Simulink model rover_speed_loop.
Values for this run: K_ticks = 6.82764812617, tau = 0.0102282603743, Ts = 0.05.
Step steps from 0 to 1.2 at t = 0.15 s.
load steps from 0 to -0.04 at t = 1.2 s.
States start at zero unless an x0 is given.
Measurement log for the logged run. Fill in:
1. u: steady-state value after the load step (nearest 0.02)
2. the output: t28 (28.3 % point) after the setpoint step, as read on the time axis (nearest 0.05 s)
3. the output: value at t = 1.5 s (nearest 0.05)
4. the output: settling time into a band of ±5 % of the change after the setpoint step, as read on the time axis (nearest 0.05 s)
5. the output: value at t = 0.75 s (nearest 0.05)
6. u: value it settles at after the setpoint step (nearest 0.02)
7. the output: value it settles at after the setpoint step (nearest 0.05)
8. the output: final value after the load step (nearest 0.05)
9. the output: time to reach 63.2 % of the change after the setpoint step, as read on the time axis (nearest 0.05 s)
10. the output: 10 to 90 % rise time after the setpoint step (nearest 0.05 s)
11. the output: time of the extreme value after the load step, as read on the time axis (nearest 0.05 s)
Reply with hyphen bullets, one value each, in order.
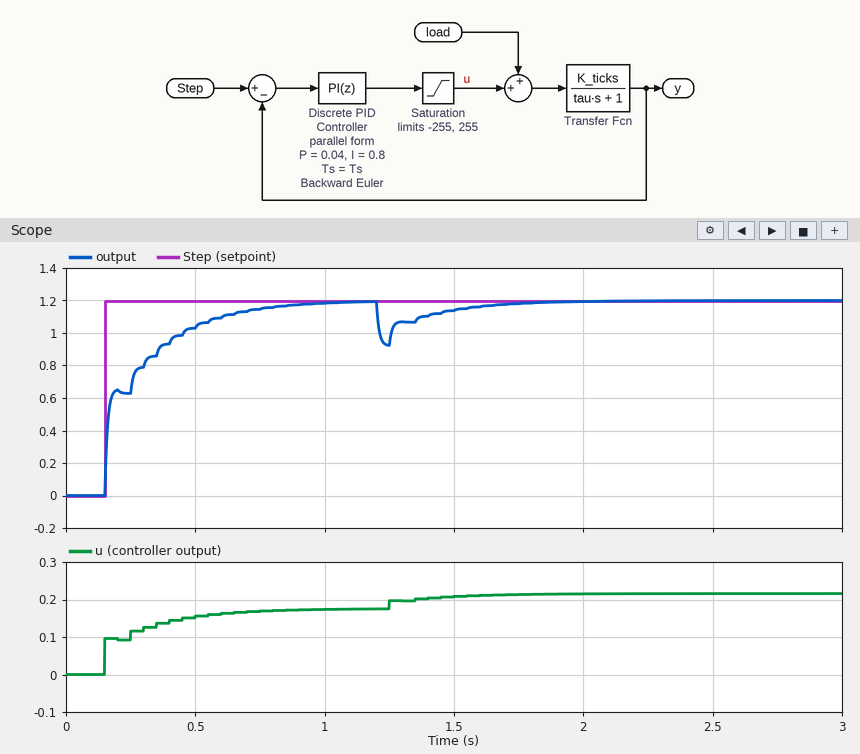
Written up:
- 0.22
- 0.15 s
- 1.15
- 0.70 s
- 1.15
- 0.18
- 1.20
- 1.20
- 0.25 s
- 0.40 s
- 1.25 s
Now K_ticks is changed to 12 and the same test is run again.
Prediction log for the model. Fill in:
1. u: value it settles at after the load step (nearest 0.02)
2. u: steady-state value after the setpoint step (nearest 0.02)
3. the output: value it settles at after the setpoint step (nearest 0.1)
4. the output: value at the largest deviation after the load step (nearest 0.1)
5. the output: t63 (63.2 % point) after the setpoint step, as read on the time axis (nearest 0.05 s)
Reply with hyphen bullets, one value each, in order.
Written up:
- 0.14
- 0.10
- 1.2
- 0.7
- 0.15 s
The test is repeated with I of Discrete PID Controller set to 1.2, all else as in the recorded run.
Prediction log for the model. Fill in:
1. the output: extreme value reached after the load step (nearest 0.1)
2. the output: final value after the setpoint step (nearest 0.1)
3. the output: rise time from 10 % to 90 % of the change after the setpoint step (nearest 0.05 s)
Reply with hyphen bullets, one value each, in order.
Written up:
- 0.9
- 1.2
- 0.25 s
